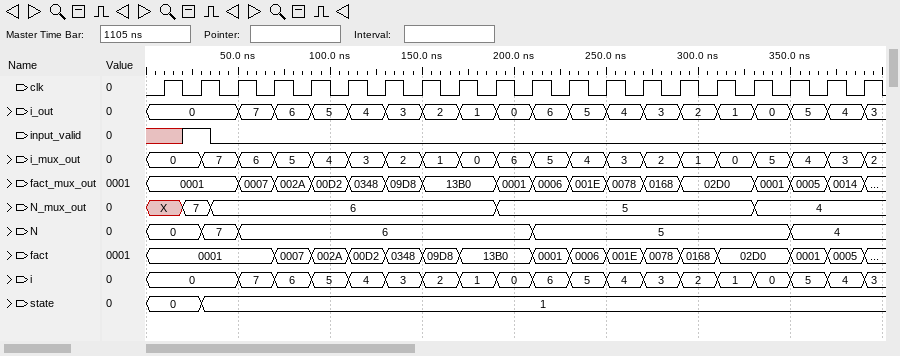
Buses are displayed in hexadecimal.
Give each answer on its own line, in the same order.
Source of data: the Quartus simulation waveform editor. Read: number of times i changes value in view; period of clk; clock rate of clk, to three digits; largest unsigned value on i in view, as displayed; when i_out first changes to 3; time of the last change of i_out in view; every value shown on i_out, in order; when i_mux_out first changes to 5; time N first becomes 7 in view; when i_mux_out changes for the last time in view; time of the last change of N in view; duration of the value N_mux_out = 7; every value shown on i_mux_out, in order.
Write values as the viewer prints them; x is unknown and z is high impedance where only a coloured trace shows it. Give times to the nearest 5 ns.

18
20 ns
50.0 MHz
7
130 ns
390 ns
0, 7, 6, 5, 4, 3, 2, 1, 0, 6, 5, 4, 3, 2, 1, 0, 5, 4, 3
70 ns
30 ns
390 ns
350 ns
15 ns
0, 7, 6, 5, 4, 3, 2, 1, 0, 6, 5, 4, 3, 2, 1, 0, 5, 4, 3, 2
